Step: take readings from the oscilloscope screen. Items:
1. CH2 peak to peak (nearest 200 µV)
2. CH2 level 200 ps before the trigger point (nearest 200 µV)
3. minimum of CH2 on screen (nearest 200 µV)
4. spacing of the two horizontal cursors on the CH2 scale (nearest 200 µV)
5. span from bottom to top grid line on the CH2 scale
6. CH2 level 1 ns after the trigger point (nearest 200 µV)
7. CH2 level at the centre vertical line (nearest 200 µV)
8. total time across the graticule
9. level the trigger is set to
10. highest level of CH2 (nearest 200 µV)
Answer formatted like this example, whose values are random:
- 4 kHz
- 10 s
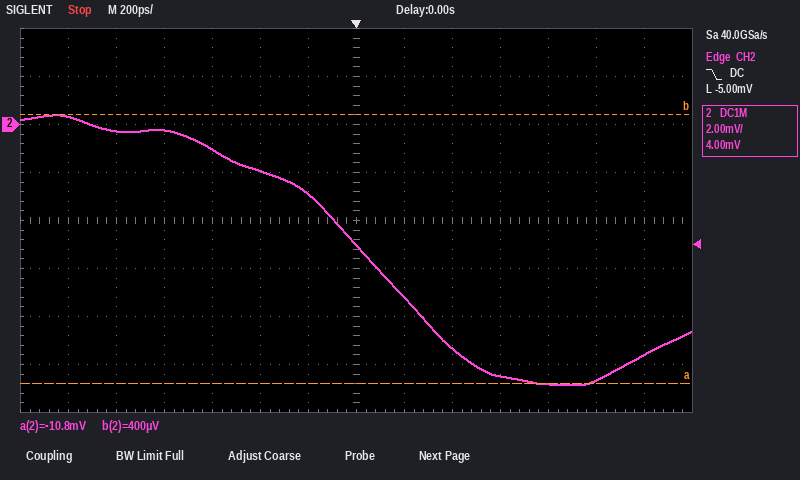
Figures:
- 11.2 mV
- -2.8 mV
- -10.8 mV
- 11.2 mV
- 16 mV
- -10.6 mV
- -5.0 mV
- 2.8 ns
- -5.00 mV
- 400 µV
